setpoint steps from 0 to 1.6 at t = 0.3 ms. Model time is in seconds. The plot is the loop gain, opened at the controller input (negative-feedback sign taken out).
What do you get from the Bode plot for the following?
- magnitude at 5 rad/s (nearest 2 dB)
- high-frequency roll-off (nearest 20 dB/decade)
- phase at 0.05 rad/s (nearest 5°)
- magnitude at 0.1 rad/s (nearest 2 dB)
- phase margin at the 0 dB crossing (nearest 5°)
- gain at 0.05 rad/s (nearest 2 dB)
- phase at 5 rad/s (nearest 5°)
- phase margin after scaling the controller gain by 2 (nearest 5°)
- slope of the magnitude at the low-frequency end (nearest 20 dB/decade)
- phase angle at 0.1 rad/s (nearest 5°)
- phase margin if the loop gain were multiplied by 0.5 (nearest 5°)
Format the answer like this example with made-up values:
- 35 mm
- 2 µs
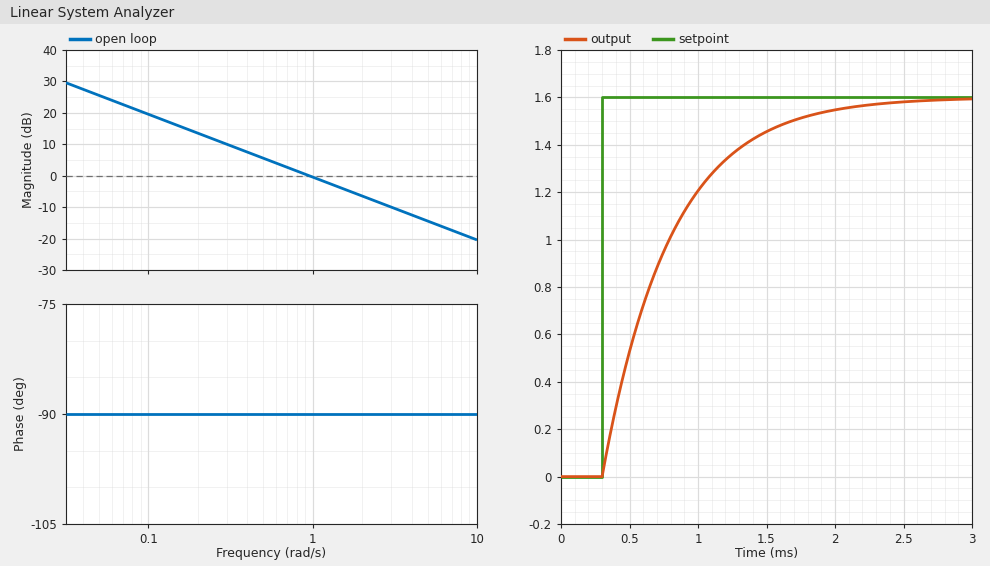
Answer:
- -14 dB
- -20 dB/decade
- -90°
- 20 dB
- 90°
- 26 dB
- -90°
- 90°
- -20 dB/decade
- -90°
- 90°
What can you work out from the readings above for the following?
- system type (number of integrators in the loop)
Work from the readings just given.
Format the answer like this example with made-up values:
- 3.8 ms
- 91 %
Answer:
- 1
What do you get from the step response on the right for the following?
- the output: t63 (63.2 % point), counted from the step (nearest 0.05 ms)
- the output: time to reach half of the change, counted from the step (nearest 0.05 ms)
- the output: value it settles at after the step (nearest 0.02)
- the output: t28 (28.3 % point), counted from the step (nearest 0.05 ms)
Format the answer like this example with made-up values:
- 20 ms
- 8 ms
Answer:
- 0.50 ms
- 0.35 ms
- 1.60
- 0.15 ms
